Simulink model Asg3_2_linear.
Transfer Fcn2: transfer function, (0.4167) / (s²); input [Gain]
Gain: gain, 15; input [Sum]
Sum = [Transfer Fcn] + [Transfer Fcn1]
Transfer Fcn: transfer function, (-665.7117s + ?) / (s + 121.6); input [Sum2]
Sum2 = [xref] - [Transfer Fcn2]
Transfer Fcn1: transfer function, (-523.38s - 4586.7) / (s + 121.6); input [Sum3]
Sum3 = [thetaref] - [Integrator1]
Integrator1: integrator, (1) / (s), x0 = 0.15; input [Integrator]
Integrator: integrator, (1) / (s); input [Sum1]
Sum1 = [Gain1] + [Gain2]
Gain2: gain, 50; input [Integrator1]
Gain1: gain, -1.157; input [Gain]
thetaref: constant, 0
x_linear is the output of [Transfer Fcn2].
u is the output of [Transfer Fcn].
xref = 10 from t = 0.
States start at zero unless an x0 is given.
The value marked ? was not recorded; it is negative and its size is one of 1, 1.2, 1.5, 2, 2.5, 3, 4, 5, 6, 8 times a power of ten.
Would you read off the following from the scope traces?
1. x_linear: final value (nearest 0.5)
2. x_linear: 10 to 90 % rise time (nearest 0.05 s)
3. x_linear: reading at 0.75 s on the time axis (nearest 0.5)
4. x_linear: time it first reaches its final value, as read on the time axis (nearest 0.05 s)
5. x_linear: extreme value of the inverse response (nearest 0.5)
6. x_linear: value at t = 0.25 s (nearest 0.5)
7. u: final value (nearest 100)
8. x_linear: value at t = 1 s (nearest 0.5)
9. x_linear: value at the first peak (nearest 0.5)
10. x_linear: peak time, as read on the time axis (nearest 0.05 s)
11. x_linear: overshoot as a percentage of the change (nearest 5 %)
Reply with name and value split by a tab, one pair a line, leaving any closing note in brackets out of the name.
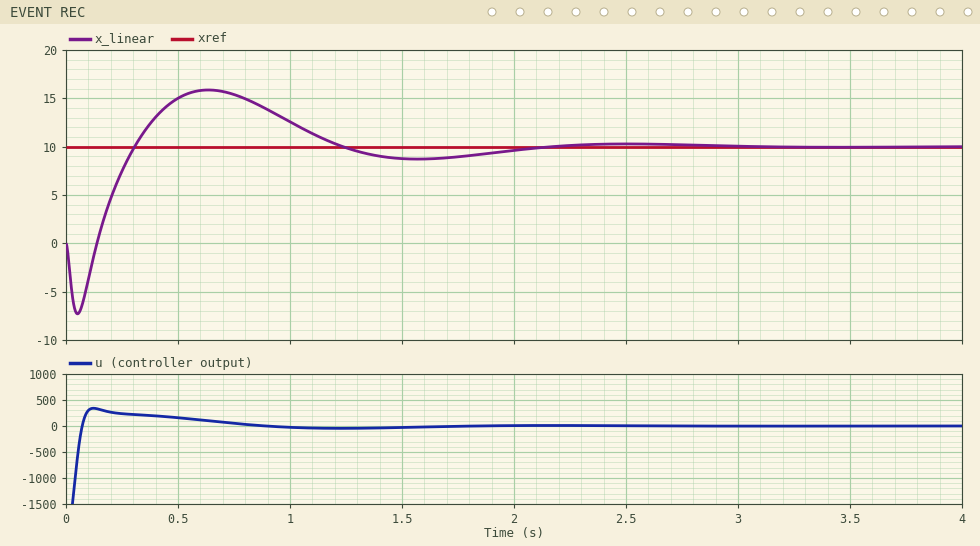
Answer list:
x_linear: final value	10.0
x_linear: 10 to 90 % rise time	0.15 s
x_linear: reading at 0.75 s on the time axis	15.5
x_linear: time it first reaches its final value, as read on the time axis	0.30 s
x_linear: extreme value of the inverse response	-7.5
x_linear: value at t = 0.25 s	7.5
u: final value	0
x_linear: value at t = 1 s	12.5
x_linear: value at the first peak	16.0
x_linear: peak time, as read on the time axis	0.65 s
x_linear: overshoot as a percentage of the change	60 %
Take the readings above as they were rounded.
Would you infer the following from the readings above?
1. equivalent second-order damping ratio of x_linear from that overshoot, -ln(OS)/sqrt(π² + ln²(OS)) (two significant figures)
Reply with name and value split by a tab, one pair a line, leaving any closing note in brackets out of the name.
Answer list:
equivalent second-order damping ratio of x_linear from that overshoot, -ln(OS)/sqrt(π² + ln²(OS))	0.16
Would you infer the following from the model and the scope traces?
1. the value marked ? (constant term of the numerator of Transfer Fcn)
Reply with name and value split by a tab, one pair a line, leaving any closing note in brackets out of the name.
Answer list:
the value marked ?	-2000
